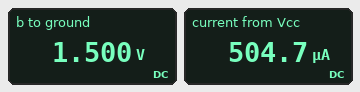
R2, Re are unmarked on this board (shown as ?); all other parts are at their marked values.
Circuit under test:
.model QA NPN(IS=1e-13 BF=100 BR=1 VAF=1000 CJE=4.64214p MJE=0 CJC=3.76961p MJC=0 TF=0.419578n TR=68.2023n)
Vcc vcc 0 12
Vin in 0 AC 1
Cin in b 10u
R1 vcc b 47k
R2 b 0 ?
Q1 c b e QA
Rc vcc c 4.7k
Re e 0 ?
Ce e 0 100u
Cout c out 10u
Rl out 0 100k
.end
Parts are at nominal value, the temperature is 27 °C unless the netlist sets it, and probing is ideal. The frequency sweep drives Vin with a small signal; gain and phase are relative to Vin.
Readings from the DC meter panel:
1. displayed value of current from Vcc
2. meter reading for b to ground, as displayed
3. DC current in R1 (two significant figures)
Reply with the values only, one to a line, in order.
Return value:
504.7 µA
1.500 V
220 µA
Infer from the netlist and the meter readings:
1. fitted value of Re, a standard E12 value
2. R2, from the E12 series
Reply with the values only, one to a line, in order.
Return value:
3.3 kΩ
6.8 kΩ
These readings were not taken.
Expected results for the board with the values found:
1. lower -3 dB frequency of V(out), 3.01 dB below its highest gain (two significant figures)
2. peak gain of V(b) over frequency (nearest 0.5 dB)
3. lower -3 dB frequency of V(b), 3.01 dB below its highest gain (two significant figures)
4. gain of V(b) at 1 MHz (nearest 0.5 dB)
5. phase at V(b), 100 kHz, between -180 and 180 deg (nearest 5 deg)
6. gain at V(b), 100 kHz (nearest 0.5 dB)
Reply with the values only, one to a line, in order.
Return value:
20 Hz
0 dB
3.1 Hz
0 dB
0 deg
0 dB
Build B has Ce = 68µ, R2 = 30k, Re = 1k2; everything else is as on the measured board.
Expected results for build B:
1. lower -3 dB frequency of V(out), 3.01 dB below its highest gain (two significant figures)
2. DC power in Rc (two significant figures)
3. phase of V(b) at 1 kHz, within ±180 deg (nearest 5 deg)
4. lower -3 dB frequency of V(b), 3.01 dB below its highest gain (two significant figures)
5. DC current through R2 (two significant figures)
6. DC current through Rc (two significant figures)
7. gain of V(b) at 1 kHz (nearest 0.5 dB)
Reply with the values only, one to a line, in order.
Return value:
740 Hz
19 mW
30 deg
730 Hz
100 µA
2.0 mA
-2.0 dB
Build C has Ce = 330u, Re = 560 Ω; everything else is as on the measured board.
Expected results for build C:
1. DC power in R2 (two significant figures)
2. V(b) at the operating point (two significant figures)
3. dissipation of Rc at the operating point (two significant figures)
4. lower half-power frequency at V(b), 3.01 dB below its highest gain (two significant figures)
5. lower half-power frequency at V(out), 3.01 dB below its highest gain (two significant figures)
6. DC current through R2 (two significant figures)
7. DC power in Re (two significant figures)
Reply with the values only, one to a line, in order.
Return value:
300 µW
1.4 V
10 mW
5.8 Hz
38 Hz
210 µA
1.2 mW
